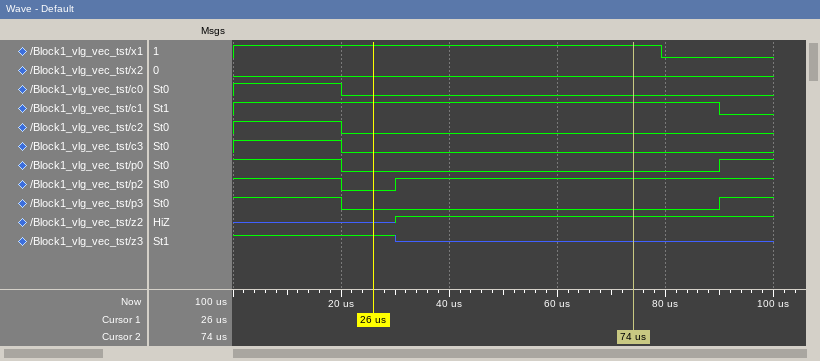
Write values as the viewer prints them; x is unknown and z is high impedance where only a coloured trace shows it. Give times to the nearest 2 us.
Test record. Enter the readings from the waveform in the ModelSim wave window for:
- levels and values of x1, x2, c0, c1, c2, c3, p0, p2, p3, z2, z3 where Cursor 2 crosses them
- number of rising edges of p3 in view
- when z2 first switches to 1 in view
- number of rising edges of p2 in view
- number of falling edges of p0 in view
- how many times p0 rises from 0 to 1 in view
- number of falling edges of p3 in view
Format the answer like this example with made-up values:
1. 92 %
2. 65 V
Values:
1. x1=1, x2=0, c0=0, c1=1, c2=0, c3=0, p0=0, p2=1, p3=0, z2=1, z3=z
2. 1
3. 30 us
4. 1
5. 1
6. 1
7. 1
